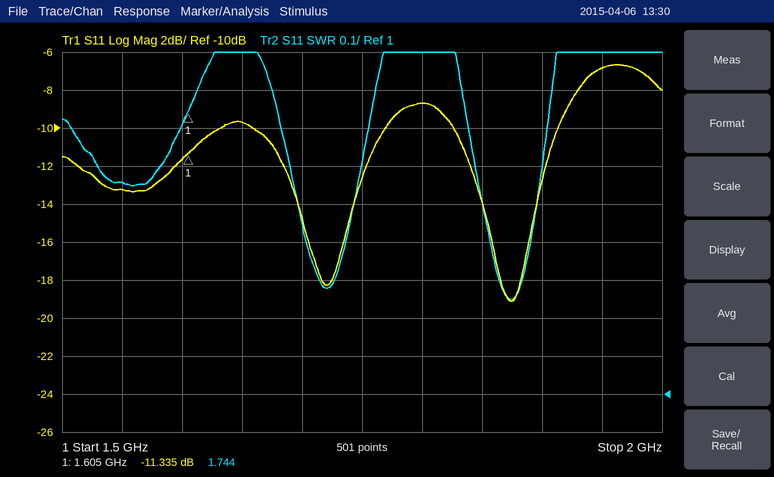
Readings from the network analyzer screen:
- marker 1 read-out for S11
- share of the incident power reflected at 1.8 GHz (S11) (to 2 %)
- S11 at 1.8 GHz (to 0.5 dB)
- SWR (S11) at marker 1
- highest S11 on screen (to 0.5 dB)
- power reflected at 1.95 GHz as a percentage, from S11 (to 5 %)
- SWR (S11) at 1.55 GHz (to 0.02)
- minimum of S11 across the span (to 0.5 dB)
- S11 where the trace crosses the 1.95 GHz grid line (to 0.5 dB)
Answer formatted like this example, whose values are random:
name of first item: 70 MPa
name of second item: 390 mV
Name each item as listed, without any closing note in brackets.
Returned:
marker 1 read-out for S11: -11.335 dB
share of the incident power reflected at 1.8 GHz (S11): 14 %
S11 at 1.8 GHz: -8.5 dB
SWR (S11) at marker 1: 1.744
highest S11 on screen: -6.5 dB
power reflected at 1.95 GHz as a percentage, from S11: 20 %
SWR (S11) at 1.55 GHz: 1.56
minimum of S11 across the span: -19.0 dB
S11 where the trace crosses the 1.95 GHz grid line: -7.0 dB
